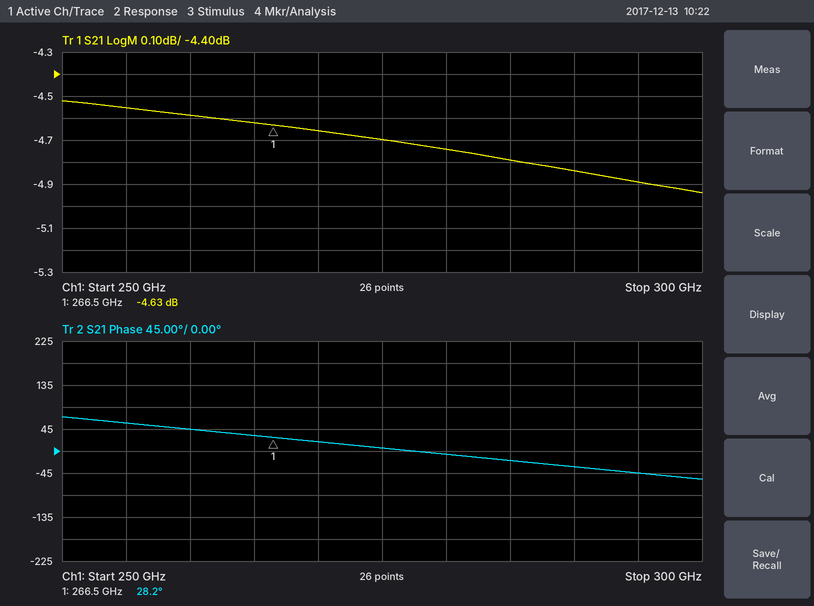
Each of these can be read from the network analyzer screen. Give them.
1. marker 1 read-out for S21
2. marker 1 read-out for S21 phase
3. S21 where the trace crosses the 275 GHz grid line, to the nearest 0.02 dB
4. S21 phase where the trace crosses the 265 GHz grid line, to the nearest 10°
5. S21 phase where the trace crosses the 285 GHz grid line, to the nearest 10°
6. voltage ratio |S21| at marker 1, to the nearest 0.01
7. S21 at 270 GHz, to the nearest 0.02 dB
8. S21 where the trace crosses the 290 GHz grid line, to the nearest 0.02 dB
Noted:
-4.63 dB
28.2°
-4.70 dB
30°
-20°
0.59
-4.66 dB
-4.84 dB
